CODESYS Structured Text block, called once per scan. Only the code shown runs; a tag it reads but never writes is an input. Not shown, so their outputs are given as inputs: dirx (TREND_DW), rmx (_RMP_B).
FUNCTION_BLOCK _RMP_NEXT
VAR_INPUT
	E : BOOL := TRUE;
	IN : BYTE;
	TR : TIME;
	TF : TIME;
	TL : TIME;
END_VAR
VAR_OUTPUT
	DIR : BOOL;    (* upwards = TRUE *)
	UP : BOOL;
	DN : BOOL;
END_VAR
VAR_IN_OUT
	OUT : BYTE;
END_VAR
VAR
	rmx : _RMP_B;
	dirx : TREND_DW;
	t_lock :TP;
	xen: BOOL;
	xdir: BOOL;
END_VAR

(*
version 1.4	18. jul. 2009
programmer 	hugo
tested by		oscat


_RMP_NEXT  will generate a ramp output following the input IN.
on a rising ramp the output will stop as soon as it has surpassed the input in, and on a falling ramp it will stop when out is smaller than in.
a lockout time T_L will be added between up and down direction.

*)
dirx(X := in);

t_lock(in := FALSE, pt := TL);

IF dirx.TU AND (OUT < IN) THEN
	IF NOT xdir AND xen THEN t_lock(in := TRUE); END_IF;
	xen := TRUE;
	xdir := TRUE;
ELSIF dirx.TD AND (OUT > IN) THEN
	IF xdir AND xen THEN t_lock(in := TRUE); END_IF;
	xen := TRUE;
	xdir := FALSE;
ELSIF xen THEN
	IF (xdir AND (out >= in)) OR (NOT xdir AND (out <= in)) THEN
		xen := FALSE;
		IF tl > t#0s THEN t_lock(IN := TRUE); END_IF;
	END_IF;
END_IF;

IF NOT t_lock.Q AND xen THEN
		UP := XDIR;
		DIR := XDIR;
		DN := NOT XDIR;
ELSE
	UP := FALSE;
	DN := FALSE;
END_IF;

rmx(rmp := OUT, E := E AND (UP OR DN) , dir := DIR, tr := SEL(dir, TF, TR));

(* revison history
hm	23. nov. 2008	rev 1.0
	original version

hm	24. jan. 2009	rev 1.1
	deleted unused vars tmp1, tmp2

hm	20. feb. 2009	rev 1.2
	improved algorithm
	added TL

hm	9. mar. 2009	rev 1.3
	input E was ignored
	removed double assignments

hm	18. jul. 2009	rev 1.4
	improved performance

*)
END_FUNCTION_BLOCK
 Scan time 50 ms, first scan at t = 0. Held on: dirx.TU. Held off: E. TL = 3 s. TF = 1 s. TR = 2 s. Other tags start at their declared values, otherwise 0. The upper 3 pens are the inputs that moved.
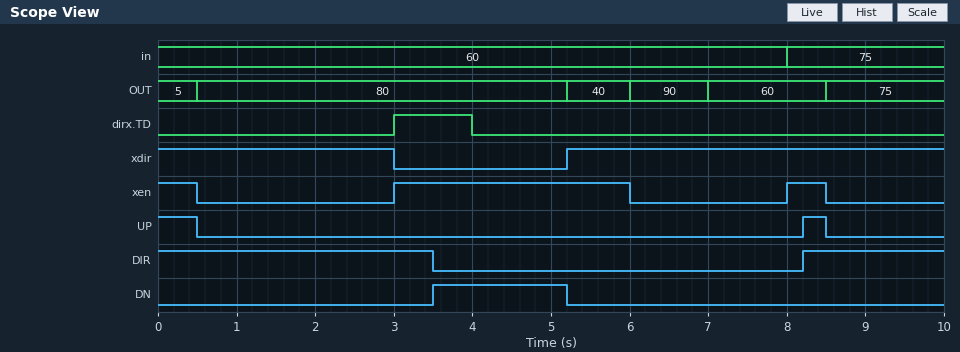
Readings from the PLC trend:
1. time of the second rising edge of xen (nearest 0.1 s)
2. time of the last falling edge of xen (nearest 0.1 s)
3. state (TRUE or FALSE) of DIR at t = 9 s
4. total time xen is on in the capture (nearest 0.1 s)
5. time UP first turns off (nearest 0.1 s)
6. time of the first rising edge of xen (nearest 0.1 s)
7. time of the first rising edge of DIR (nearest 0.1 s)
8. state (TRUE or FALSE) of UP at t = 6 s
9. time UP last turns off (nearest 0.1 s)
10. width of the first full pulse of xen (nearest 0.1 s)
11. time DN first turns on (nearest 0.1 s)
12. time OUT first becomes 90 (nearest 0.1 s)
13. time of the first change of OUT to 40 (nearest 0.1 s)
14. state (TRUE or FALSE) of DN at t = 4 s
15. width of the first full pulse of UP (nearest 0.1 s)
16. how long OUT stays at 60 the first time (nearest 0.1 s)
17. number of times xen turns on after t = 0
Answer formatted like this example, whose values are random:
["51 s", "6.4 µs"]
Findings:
["8.0 s", "8.5 s", "TRUE", "4.0 s", "0.5 s", "3.0 s", "8.2 s", "FALSE", "8.5 s", "3.0 s", "3.5 s", "6.0 s", "5.2 s", "TRUE", "0.3 s", "1.5 s", "2"]
